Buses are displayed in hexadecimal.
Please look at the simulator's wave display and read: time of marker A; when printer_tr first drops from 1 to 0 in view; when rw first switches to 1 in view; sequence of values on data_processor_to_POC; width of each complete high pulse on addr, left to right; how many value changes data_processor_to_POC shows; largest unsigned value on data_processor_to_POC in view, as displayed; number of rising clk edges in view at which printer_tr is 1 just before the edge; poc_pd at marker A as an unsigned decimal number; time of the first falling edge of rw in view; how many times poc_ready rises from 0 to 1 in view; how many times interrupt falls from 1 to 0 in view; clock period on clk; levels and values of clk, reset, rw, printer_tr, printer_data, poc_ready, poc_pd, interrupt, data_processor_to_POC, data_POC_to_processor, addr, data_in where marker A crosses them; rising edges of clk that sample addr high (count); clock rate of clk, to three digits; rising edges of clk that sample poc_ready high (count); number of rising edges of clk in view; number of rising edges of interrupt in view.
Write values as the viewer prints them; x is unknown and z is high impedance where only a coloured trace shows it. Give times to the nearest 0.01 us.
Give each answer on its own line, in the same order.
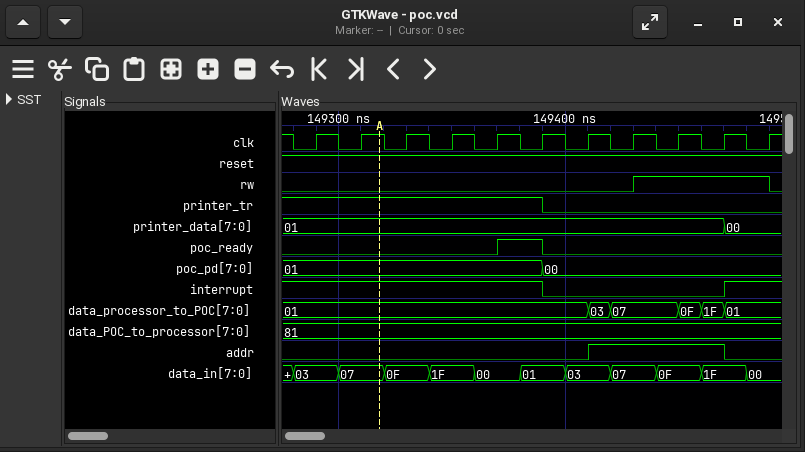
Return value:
149.32 us
149.39 us
149.43 us
01, 03, 07, 0F, 1F, 01
0.06 us
5
1F
6
1
149.49 us
1
1
0.02 us
clk=1, reset=1, rw=0, printer_tr=1, printer_data=01, poc_ready=0, poc_pd=01, interrupt=1, data_processor_to_POC=01, data_POC_to_processor=81, addr=0, data_in=07
3
50.0 MHz
1
11
1
